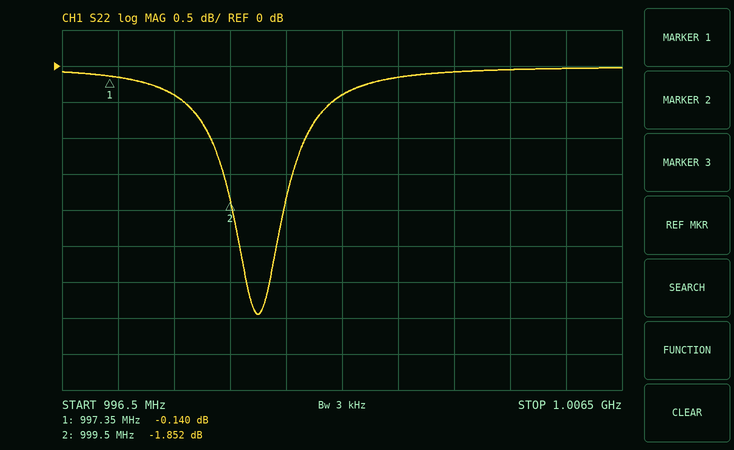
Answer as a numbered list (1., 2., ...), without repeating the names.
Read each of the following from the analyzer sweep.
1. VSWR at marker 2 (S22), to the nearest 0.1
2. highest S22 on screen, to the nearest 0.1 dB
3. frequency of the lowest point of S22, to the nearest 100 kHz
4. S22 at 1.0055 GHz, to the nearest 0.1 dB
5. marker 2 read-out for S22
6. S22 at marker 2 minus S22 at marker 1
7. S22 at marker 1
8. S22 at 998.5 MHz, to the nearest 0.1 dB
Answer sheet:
1. 9.4
2. 0.0 dB
3. 1.0000 GHz
4. 0.0 dB
5. -1.852 dB
6. -1.712 dB
7. -0.140 dB
8. -0.4 dB
